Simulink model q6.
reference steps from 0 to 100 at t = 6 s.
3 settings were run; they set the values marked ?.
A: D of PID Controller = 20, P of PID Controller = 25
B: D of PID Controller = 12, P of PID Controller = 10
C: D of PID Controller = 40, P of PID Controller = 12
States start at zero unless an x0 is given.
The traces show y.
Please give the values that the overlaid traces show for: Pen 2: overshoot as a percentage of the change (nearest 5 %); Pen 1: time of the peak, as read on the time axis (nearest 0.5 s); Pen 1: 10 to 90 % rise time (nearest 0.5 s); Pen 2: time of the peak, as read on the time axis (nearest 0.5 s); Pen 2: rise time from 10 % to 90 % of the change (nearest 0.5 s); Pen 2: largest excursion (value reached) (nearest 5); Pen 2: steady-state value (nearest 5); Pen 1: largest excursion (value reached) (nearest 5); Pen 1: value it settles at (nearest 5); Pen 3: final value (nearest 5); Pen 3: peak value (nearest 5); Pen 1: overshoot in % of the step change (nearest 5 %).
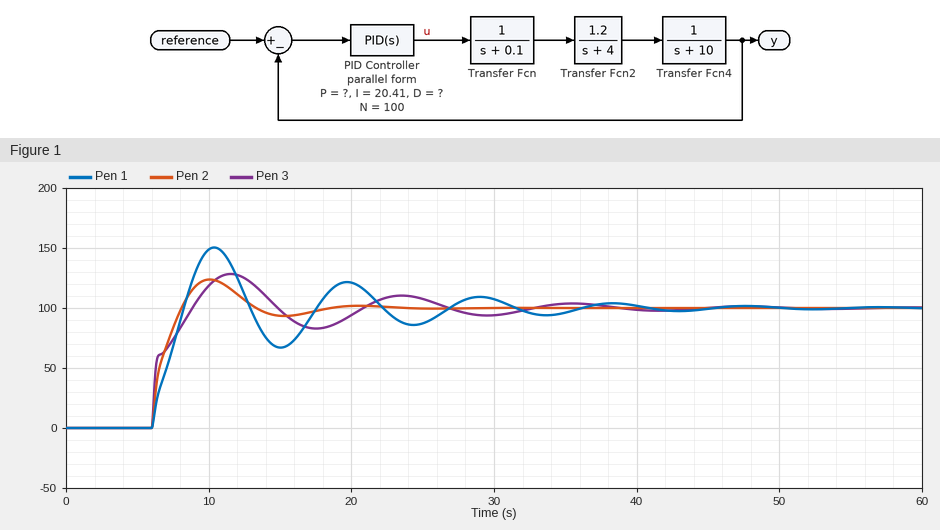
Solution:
25 %
10.5 s
2.0 s
10.0 s
1.5 s
125
100
150
100
100
130
50 %
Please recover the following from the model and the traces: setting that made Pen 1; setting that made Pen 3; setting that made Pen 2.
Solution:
B
C
A
